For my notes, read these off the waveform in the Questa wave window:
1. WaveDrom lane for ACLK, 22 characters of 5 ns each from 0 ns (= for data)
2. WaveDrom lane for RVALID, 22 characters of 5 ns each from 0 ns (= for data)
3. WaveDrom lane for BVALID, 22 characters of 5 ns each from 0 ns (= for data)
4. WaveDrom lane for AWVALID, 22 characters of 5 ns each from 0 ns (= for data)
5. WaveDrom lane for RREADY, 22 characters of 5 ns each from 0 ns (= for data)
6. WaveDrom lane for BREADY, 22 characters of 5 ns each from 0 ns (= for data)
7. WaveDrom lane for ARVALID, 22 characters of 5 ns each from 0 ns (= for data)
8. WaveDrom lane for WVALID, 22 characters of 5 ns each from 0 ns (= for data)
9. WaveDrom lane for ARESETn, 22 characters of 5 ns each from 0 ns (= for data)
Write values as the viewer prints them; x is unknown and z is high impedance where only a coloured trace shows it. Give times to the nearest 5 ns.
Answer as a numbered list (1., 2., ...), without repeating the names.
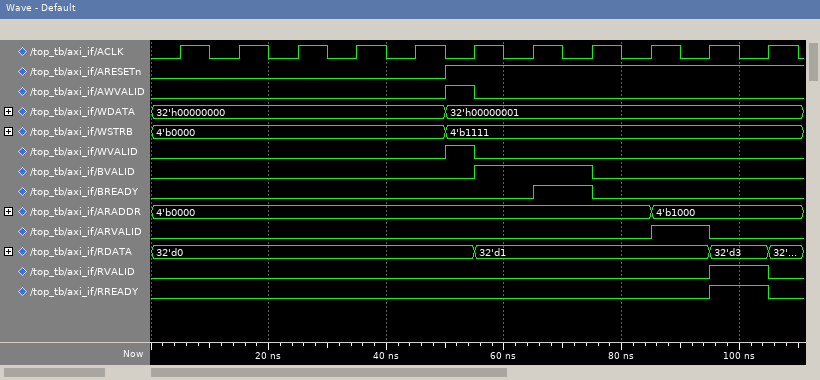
1. {name: 'ACLK', wave: '0101010101010101010101'}
2. {name: 'RVALID', wave: '0..................1.0'}
3. {name: 'BVALID', wave: '0..........1...0......'}
4. {name: 'AWVALID', wave: '0.........10..........'}
5. {name: 'RREADY', wave: '0..................1.0'}
6. {name: 'BREADY', wave: '0............1.0......'}
7. {name: 'ARVALID', wave: '0................1.0..'}
8. {name: 'WVALID', wave: '0.........10..........'}
9. {name: 'ARESETn', wave: '0.........1...........'}
